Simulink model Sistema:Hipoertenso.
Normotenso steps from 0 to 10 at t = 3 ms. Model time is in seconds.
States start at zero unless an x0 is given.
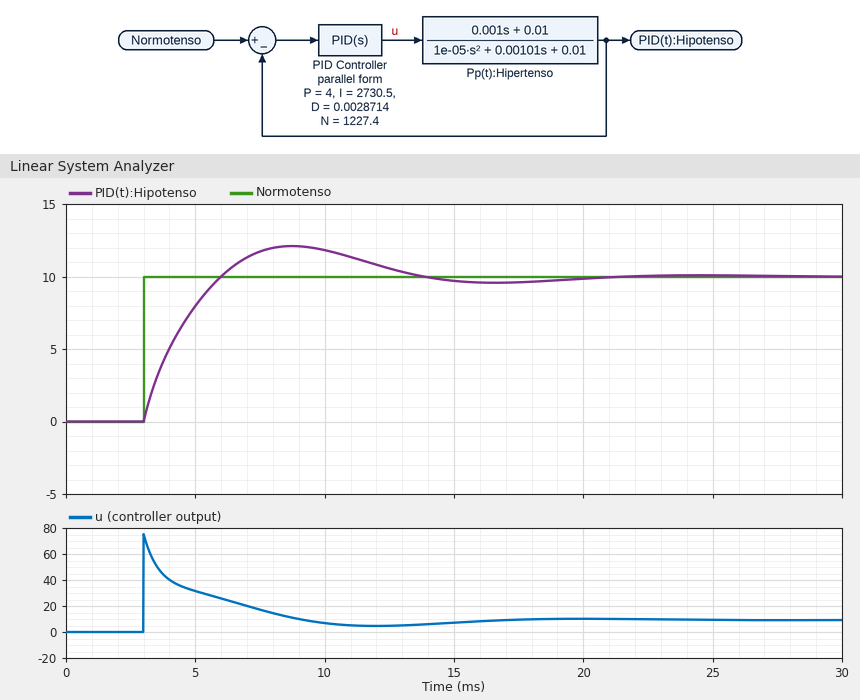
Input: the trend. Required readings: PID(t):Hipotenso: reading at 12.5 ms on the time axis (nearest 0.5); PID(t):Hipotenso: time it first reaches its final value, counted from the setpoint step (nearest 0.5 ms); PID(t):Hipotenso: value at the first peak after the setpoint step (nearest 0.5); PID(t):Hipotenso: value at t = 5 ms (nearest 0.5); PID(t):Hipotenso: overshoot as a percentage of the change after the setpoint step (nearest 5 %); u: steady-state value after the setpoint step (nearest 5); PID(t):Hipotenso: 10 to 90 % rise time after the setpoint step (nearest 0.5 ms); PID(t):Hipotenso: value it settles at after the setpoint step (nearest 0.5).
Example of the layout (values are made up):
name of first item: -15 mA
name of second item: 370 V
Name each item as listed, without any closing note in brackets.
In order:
PID(t):Hipotenso: reading at 12.5 ms on the time axis: 10.5
PID(t):Hipotenso: time it first reaches its final value, counted from the setpoint step: 3.0 ms
PID(t):Hipotenso: value at the first peak after the setpoint step: 12.0
PID(t):Hipotenso: value at t = 5 ms: 8.0
PID(t):Hipotenso: overshoot as a percentage of the change after the setpoint step: 20 %
u: steady-state value after the setpoint step: 10
PID(t):Hipotenso: 10 to 90 % rise time after the setpoint step: 2.5 ms
PID(t):Hipotenso: value it settles at after the setpoint step: 10.0
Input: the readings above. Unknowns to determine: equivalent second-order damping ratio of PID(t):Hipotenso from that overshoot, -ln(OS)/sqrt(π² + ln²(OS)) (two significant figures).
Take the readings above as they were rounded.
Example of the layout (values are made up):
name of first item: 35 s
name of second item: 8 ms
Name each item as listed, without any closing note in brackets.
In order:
equivalent second-order damping ratio of PID(t):Hipotenso from that overshoot, -ln(OS)/sqrt(π² + ln²(OS)): 0.46
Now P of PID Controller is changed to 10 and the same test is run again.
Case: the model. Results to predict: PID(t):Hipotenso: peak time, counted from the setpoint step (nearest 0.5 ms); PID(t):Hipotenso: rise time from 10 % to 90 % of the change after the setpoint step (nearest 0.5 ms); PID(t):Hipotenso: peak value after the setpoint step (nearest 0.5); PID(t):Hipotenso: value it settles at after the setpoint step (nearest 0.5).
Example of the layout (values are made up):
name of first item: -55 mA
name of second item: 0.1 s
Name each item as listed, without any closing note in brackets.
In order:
PID(t):Hipotenso: peak time, counted from the setpoint step: 5.0 ms
PID(t):Hipotenso: rise time from 10 % to 90 % of the change after the setpoint step: 1.5 ms
PID(t):Hipotenso: peak value after the setpoint step: 10.5
PID(t):Hipotenso: value it settles at after the setpoint step: 10.0
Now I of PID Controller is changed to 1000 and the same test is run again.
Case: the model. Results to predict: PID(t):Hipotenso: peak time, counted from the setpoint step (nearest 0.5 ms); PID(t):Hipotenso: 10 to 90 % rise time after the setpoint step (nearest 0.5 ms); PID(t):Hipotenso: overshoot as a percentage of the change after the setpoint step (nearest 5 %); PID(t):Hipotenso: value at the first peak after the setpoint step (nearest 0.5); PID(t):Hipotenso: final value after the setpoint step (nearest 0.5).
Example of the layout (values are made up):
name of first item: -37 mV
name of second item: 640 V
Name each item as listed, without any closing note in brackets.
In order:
PID(t):Hipotenso: peak time, counted from the setpoint step: 9.5 ms
PID(t):Hipotenso: 10 to 90 % rise time after the setpoint step: 4.0 ms
PID(t):Hipotenso: overshoot as a percentage of the change after the setpoint step: 10 %
PID(t):Hipotenso: value at the first peak after the setpoint step: 11.0
PID(t):Hipotenso: final value after the setpoint step: 10.0
